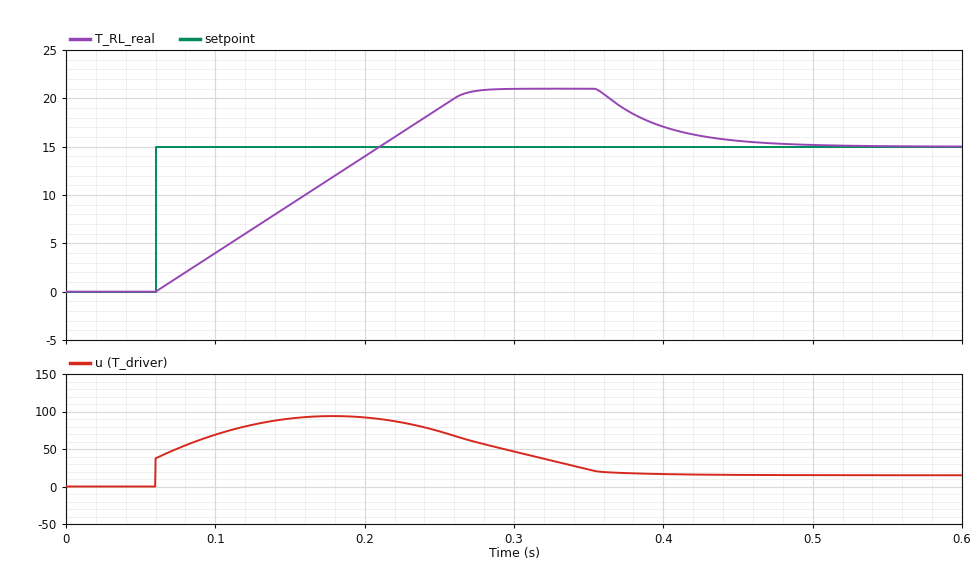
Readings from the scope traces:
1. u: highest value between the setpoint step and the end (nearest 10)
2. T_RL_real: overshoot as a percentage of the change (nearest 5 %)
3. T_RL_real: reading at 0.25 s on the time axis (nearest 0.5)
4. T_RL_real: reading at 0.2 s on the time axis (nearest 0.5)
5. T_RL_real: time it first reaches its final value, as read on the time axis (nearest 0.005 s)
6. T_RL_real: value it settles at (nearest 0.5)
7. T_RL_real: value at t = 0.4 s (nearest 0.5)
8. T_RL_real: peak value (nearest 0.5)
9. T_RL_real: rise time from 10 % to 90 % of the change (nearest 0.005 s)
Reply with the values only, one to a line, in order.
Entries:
90
40 %
19.0
14.0
0.210 s
15.0
17.0
21.0
0.120 s
